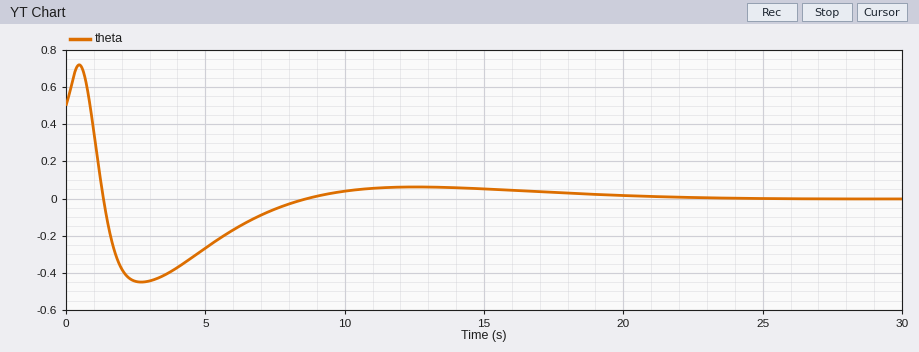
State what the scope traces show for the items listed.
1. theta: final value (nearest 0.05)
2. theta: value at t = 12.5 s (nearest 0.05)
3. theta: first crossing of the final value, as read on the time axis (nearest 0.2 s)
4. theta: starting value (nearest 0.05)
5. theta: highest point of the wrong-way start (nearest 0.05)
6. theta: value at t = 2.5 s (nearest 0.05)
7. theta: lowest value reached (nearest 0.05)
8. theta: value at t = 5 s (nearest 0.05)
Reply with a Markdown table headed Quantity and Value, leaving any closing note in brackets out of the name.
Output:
| Quantity | Value |
|---|---|
| theta: final value | 0.00 |
| theta: value at t = 12.5 s | 0.05 |
| theta: first crossing of the final value, as read on the time axis | 1.4 s |
| theta: starting value | 0.50 |
| theta: highest point of the wrong-way start | 0.70 |
| theta: value at t = 2.5 s | -0.45 |
| theta: lowest value reached | -0.45 |
| theta: value at t = 5 s | -0.25 |
